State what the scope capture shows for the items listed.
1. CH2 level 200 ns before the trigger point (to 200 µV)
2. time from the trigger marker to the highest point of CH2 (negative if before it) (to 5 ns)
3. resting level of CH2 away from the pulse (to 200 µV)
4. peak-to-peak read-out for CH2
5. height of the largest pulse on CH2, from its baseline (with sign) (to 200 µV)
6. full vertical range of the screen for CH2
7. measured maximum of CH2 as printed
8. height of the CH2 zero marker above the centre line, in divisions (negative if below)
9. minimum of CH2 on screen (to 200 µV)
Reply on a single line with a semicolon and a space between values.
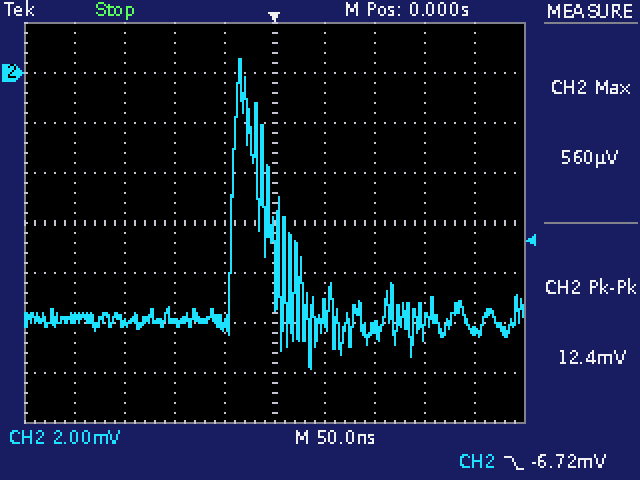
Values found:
-9.8 mV; -35 ns; -9.8 mV; 12.4 mV; +10.4 mV; 16 mV; 560 µV; +3.0 div; -11.8 mV
